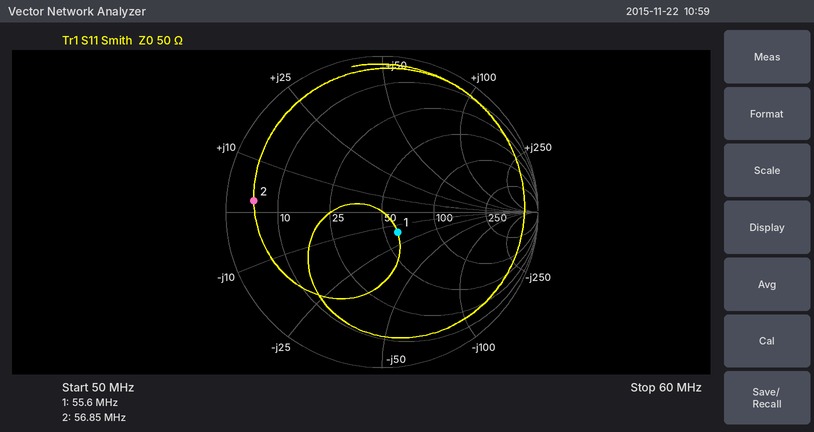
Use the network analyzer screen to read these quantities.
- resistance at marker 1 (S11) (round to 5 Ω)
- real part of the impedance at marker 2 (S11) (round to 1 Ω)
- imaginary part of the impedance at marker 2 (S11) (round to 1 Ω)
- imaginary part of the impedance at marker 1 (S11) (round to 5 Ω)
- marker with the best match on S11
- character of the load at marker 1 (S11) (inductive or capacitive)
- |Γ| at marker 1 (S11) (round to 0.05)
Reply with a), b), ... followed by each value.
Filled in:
a) 60 Ω
b) 5 Ω
c) +2 Ω
d) -15 Ω
e) marker 1
f) capacitive
g) 0.15
